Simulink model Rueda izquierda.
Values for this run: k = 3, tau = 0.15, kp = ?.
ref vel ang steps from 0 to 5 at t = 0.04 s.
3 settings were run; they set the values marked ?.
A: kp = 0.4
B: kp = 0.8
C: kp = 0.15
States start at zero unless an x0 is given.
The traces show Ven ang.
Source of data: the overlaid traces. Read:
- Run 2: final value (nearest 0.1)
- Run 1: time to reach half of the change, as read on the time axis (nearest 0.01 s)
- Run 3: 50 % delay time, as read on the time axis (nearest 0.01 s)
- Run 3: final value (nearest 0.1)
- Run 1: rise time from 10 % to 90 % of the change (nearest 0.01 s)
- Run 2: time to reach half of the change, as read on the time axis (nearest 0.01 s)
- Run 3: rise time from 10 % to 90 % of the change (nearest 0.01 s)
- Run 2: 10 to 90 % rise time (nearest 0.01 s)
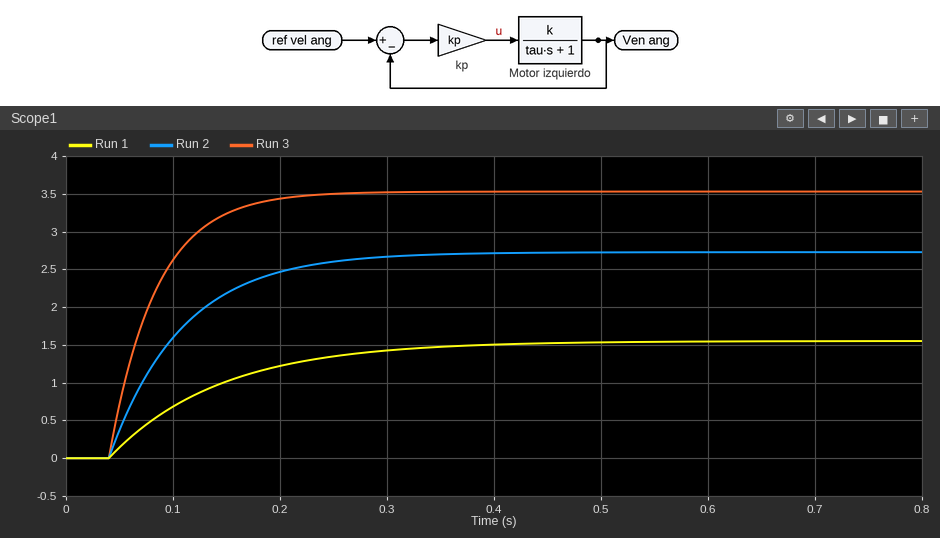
2.7
0.11 s
0.07 s
3.5
0.23 s
0.09 s
0.10 s
0.15 s
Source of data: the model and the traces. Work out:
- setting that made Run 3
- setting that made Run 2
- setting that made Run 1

B
A
C
